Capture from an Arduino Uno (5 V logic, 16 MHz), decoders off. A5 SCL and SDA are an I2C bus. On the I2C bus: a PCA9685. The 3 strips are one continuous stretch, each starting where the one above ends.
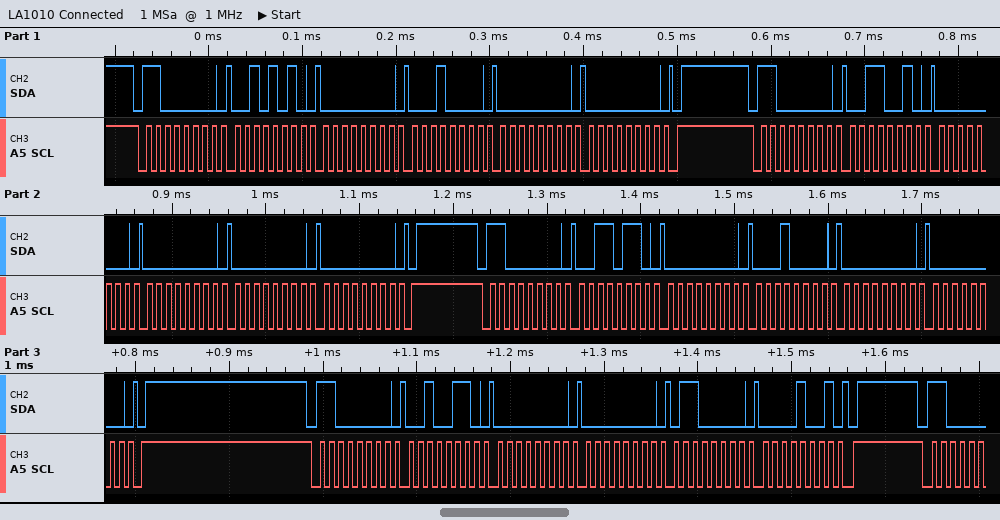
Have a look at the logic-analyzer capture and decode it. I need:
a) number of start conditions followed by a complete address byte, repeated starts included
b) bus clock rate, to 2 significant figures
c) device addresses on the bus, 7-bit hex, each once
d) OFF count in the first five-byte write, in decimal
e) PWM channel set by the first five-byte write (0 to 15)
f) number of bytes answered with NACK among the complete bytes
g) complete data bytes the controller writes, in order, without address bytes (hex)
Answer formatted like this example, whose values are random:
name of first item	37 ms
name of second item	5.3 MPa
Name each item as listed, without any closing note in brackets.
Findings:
number of start conditions followed by a complete address byte, repeated starts included	4
bus clock rate, to 2 significant figures	100 kHz
device addresses on the bus, 7-bit hex, each once	0x60
OFF count in the first five-byte write, in decimal	0
PWM channel set by the first five-byte write	9
number of bytes answered with NACK among the complete bytes	0
complete data bytes the controller writes, in order, without address bytes	2A 00 10 00 00 32 00 00 00 00 36 00 10 00 00 26 00 00 60 09
